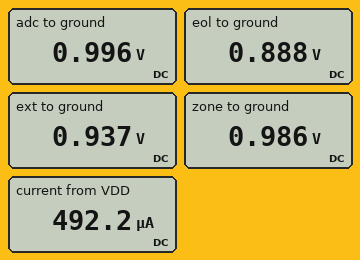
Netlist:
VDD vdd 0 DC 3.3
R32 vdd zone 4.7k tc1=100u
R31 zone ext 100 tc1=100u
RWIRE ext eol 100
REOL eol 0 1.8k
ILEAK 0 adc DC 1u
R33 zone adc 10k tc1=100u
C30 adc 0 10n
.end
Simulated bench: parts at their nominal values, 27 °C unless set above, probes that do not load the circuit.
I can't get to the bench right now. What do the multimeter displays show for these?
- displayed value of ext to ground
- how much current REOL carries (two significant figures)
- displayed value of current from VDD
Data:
0.937 V
490 µA
492.2 µA
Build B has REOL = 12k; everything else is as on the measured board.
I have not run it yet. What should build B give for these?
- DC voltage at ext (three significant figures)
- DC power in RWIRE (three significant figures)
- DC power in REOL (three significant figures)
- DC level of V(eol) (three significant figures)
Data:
2.37 V
3.82 µW
459 µW
2.35 V
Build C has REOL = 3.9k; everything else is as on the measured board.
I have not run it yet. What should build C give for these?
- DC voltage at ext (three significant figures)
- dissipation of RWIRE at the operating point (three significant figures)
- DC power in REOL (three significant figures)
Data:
1.50 V
14.1 µW
550 µW
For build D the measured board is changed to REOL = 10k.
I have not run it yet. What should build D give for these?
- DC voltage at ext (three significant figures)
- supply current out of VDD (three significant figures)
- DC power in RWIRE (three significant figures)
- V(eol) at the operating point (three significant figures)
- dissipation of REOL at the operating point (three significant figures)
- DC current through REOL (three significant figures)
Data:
2.24 V
221 µA
4.92 µW
2.22 V
492 µW
222 µA
